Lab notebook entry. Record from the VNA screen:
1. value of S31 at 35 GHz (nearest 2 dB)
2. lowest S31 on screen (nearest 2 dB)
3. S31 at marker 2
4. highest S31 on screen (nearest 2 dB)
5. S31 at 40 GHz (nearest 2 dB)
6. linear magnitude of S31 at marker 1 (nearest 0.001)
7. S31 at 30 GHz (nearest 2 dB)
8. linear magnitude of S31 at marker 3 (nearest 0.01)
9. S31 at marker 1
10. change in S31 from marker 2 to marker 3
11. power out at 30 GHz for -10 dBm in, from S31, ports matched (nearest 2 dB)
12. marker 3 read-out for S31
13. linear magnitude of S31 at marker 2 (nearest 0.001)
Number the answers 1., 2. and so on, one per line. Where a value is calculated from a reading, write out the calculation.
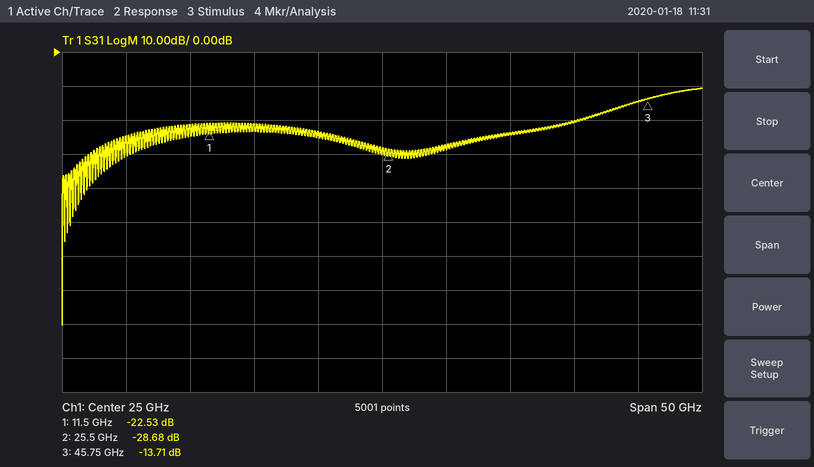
1. -24 dB
2. -80 dB
3. -28.68 dB
4. -10 dB
5. -20 dB
6. 10^(-22.53/20) ≈ 0.075
7. -28 dB
8. 10^(-13.71/20) ≈ 0.21
9. -22.53 dB
10. -13.71 − (-28.68) = 14.97 dB
11. -10 dBm + (-28 dB) = -38 dBm
12. -13.71 dB
13. 10^(-28.68/20) ≈ 0.037
